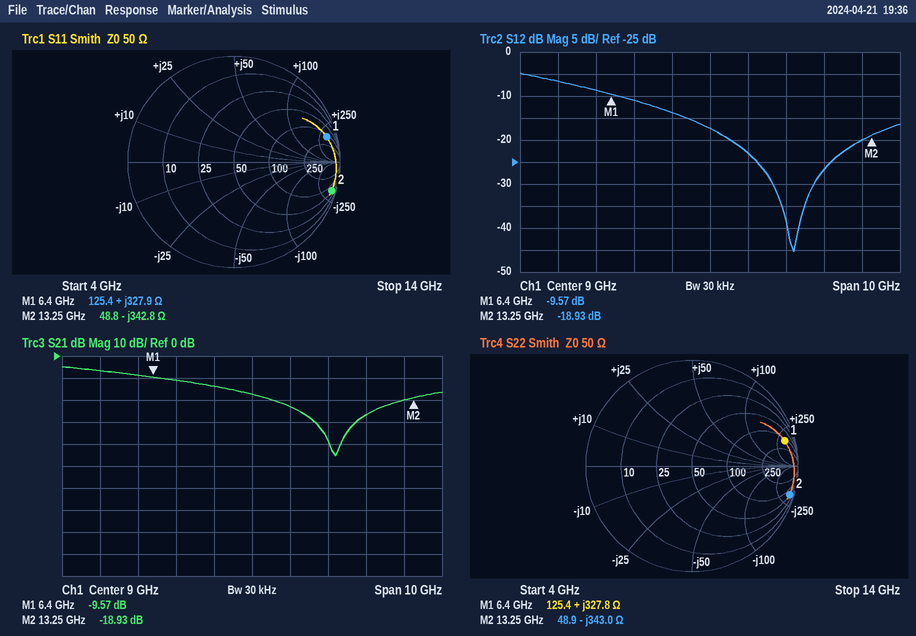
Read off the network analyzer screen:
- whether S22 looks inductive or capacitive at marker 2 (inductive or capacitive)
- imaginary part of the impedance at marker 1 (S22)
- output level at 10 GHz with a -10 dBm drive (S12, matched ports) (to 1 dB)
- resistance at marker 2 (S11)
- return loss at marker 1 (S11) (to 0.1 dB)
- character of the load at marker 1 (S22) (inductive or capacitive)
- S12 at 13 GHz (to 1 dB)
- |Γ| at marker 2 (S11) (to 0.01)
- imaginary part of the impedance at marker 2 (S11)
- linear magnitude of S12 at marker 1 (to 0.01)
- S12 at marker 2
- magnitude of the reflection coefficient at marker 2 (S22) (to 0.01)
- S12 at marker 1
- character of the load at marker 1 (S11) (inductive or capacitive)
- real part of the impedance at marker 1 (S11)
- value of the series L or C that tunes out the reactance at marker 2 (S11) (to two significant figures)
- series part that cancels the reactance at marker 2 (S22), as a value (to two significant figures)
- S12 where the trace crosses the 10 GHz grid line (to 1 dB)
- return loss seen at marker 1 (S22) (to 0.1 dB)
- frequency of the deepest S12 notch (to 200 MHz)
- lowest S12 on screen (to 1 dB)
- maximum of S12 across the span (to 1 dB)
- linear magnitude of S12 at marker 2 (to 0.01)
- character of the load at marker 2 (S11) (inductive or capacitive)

capacitive
+327.8 Ω
-33 dBm
48.8 Ω
0.9 dB
inductive
-20 dB
0.96
-342.8 Ω
0.33
-18.93 dB
0.96
-9.57 dB
inductive
125.4 Ω
4.1 nH
4.1 nH
-23 dB
0.9 dB
11.2 GHz
-45 dB
-5 dB
0.11
capacitive
